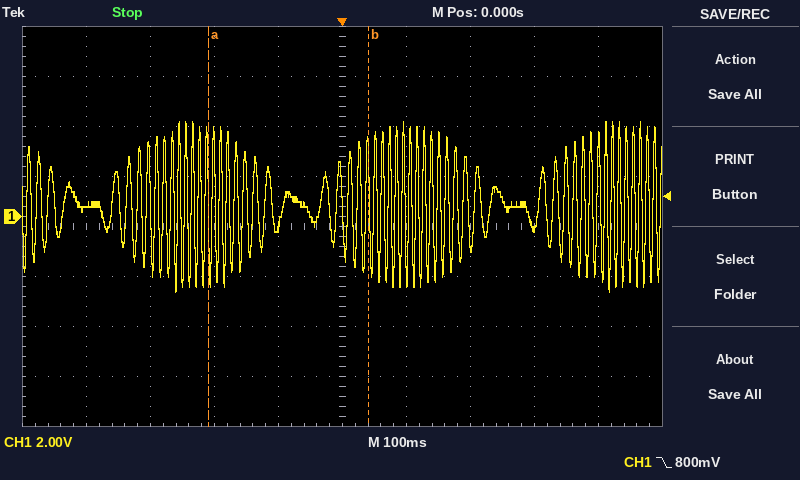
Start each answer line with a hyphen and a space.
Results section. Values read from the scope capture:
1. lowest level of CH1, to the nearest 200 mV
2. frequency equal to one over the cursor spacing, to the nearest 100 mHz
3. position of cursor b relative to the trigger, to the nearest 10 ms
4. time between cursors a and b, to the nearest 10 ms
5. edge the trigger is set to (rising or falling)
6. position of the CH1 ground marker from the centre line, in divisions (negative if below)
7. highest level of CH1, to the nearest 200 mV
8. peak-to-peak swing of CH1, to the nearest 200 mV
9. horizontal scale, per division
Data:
- -3.0 V
- 4.0 Hz
- +40 ms
- 250 ms
- falling
- +0.2 div
- 3.8 V
- 6.8 V
- 100 ms
